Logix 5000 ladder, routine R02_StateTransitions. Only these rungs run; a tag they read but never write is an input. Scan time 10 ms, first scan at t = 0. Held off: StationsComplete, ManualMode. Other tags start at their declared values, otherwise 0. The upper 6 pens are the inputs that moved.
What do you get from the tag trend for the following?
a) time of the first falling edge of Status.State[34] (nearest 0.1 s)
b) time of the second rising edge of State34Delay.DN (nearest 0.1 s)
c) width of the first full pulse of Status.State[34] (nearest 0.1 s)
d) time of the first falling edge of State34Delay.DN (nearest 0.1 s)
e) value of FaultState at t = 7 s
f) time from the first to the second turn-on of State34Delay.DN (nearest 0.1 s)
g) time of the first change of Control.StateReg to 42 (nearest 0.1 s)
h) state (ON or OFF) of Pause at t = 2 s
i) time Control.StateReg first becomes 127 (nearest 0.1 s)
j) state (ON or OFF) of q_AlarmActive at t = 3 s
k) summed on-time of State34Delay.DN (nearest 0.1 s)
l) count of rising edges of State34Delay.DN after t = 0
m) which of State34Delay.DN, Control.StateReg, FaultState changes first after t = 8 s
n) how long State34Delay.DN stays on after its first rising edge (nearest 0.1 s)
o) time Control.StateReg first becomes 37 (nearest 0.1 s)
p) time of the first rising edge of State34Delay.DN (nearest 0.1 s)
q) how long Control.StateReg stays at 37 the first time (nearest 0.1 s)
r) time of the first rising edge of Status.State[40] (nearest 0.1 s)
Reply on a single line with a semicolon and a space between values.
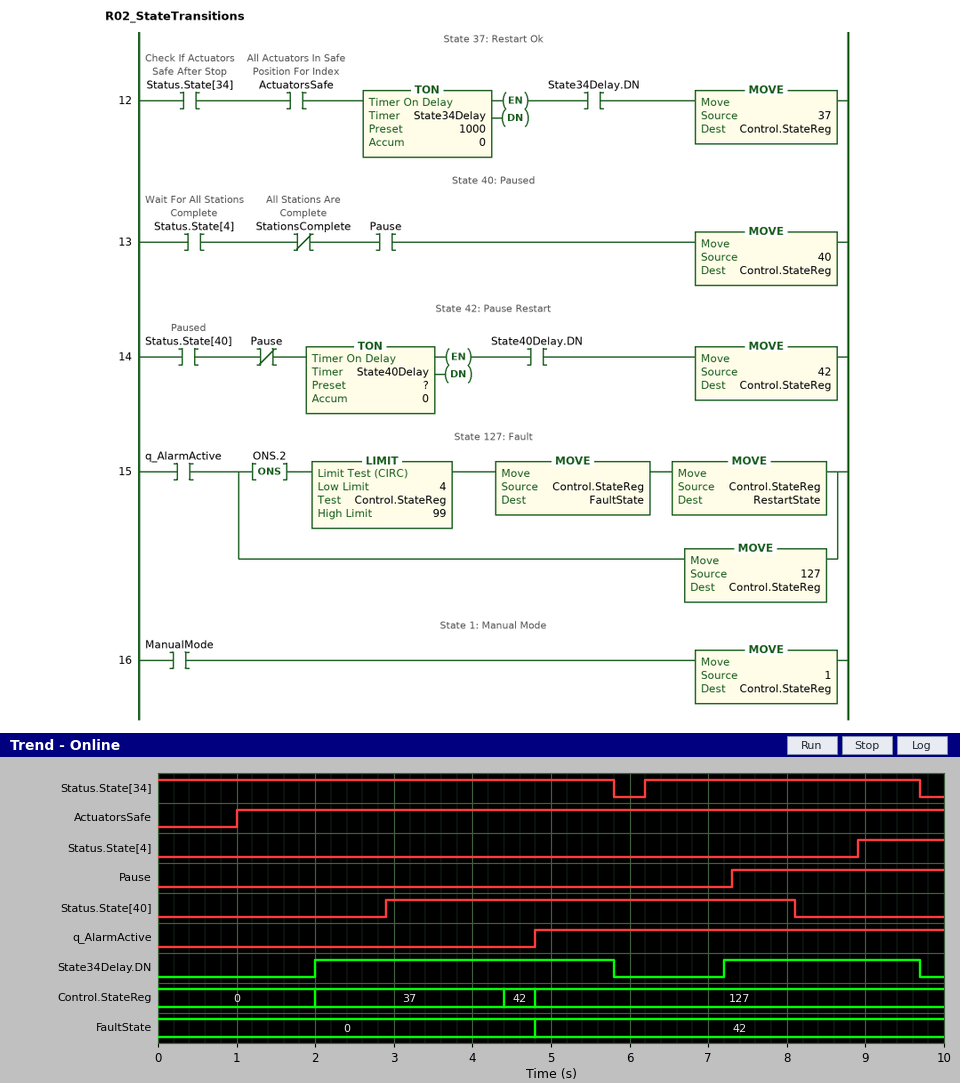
5.8 s; 7.2 s; 3.5 s; 5.8 s; 42; 5.2 s; 4.4 s; OFF; 4.8 s; OFF; 6.3 s; 2; State34Delay.DN; 3.8 s; 2.0 s; 2.0 s; 2.4 s; 2.9 s
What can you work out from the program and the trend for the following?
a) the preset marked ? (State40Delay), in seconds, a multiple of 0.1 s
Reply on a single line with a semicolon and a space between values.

1.5 s
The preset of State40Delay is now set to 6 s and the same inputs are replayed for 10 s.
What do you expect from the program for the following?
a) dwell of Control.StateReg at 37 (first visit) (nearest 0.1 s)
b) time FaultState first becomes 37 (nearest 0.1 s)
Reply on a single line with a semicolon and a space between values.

2.8 s; 4.8 s
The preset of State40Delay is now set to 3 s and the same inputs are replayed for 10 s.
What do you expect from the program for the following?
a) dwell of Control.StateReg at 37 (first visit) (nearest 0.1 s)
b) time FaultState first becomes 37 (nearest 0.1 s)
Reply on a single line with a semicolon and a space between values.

2.8 s; 4.8 s
